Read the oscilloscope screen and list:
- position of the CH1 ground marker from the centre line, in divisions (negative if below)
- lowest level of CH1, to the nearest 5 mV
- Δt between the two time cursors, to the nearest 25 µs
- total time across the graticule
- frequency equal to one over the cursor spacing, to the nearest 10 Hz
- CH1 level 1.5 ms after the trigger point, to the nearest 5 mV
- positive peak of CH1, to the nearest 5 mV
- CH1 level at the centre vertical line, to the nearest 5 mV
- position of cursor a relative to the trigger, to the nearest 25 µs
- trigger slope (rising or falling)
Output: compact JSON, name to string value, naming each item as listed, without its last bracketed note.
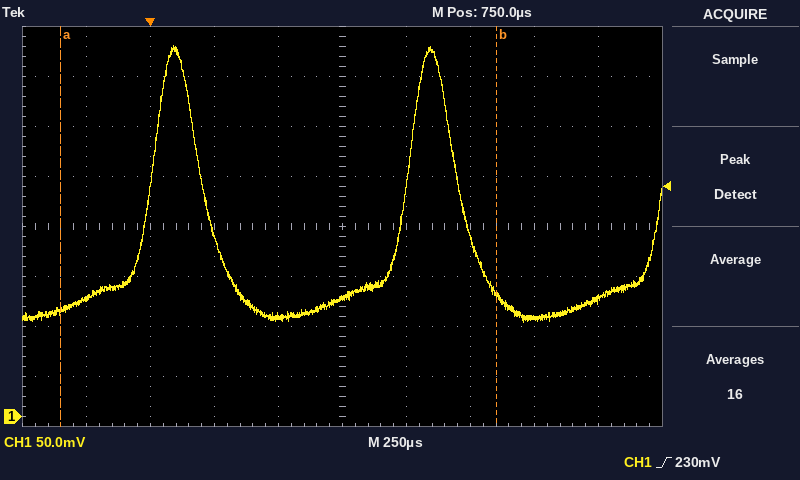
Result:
{"position of the CH1 ground marker from the centre line, in divisions": "-3.8 div", "lowest level of CH1, to the nearest 5 mV": "95 mV", "Δt between the two time cursors, to the nearest 25 µs": "1.700 ms", "total time across the graticule": "2.5 ms", "frequency equal to one over the cursor spacing, to the nearest 10 Hz": "590 Hz", "CH1 level 1.5 ms after the trigger point, to the nearest 5 mV": "100 mV", "positive peak of CH1, to the nearest 5 mV": "370 mV", "CH1 level at the centre vertical line, to the nearest 5 mV": "120 mV", "position of cursor a relative to the trigger, to the nearest 25 µs": "-350 µs", "trigger slope": "rising"}
